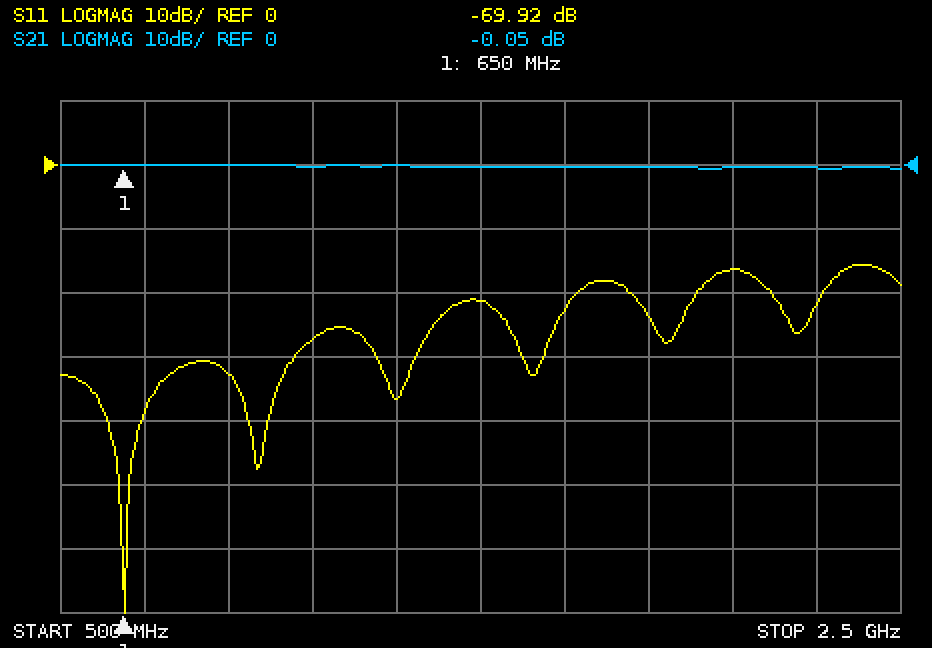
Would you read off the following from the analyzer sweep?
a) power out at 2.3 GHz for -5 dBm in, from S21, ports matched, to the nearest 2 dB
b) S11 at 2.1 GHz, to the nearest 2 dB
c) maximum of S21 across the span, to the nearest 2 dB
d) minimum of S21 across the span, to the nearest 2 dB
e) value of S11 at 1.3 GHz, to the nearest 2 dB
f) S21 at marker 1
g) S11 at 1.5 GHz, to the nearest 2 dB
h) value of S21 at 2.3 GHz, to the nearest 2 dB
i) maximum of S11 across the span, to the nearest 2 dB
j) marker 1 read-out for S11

-6 dBm
-16 dB
0 dB
0 dB
-36 dB
-0.05 dB
-22 dB
0 dB
-16 dB
-69.92 dB
